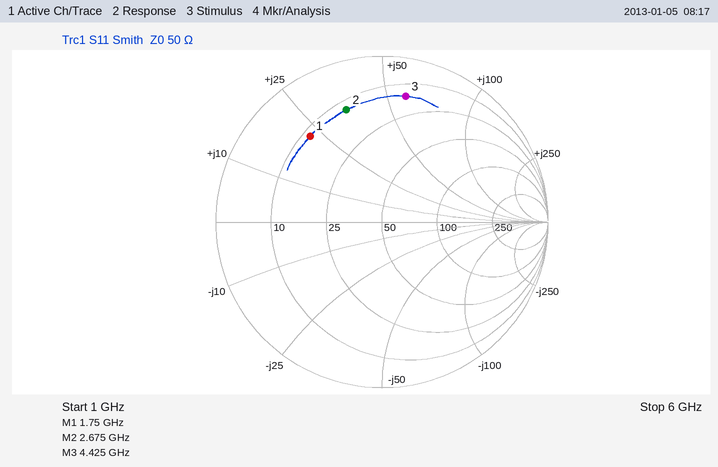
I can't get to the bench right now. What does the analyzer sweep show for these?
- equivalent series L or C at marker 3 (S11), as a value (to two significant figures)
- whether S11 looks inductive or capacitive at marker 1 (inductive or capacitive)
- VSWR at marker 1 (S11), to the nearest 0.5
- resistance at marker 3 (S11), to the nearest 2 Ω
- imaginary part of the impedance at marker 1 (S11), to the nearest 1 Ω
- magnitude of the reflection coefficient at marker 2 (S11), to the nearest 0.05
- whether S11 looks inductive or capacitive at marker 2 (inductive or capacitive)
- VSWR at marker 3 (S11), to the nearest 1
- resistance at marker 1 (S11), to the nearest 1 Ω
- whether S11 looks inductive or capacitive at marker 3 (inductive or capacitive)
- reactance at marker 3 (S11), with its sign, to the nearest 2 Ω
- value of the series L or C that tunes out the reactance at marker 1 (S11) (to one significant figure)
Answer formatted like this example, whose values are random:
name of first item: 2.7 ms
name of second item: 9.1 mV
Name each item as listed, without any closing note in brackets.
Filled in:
equivalent series L or C at marker 3 (S11), as a value: 2.1 nH
whether S11 looks inductive or capacitive at marker 1: inductive
VSWR at marker 1 (S11), to the nearest 0.5: 5.0
resistance at marker 3 (S11), to the nearest 2 Ω: 16 Ω
imaginary part of the impedance at marker 1 (S11), to the nearest 1 Ω: +22 Ω
magnitude of the reflection coefficient at marker 2 (S11), to the nearest 0.05: 0.70
whether S11 looks inductive or capacitive at marker 2: inductive
VSWR at marker 3 (S11), to the nearest 1: 8
resistance at marker 1 (S11), to the nearest 1 Ω: 12 Ω
whether S11 looks inductive or capacitive at marker 3: inductive
reactance at marker 3 (S11), with its sign, to the nearest 2 Ω: +58 Ω
value of the series L or C that tunes out the reactance at marker 1 (S11): 4 pF
